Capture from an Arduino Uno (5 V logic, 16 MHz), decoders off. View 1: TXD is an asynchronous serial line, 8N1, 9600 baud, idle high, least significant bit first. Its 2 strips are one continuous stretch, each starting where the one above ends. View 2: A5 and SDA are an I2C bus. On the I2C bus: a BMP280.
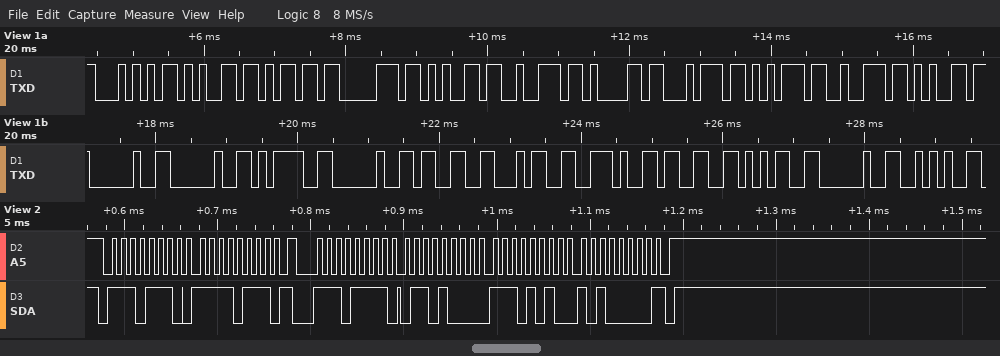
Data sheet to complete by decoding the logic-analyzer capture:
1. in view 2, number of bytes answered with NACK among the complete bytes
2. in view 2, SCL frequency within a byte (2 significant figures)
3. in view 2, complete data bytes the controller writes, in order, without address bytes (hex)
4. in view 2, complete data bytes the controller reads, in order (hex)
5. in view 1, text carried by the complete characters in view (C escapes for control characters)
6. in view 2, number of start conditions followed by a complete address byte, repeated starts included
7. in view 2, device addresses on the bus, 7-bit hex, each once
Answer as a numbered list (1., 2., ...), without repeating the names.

1. 1
2. 100 kHz
3. F7
4. 68 EA A0
5. "Temperature  = 34.35 *"
6. 2
7. 0x77
